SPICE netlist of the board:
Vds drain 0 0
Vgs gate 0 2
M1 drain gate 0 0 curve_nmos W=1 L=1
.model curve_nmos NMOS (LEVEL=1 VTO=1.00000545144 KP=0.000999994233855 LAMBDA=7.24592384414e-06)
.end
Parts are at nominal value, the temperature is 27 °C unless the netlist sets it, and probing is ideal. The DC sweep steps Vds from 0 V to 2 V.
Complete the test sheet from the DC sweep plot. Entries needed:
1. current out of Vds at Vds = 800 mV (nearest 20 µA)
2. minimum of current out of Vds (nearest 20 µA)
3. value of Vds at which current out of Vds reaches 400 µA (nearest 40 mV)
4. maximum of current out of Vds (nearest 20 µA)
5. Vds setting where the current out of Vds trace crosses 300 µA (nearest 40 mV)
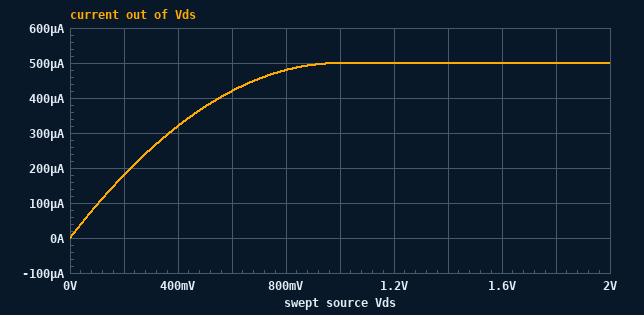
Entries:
480 µA
0 A
560 mV
500 µA
360 mV
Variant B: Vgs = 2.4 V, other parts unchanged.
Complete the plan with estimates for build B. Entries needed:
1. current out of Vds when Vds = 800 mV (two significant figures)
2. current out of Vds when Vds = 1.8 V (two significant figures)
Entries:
800 µA
980 µA
